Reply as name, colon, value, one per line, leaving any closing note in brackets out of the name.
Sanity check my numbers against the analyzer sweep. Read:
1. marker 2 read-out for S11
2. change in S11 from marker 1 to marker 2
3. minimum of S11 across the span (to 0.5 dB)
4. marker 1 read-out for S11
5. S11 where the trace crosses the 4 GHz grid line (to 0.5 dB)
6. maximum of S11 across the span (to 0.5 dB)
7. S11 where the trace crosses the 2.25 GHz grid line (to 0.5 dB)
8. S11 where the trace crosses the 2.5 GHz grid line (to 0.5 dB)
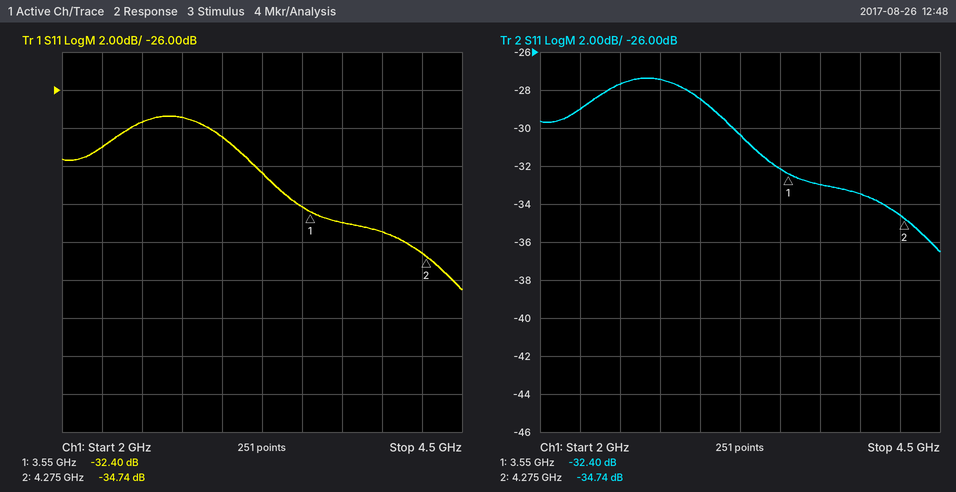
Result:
marker 2 read-out for S11: -34.74 dB
change in S11 from marker 1 to marker 2: -2.34 dB
minimum of S11 across the span: -36.5 dB
marker 1 read-out for S11: -32.40 dB
S11 where the trace crosses the 4 GHz grid line: -33.5 dB
maximum of S11 across the span: -27.5 dB
S11 where the trace crosses the 2.25 GHz grid line: -29.0 dB
S11 where the trace crosses the 2.5 GHz grid line: -27.5 dB
